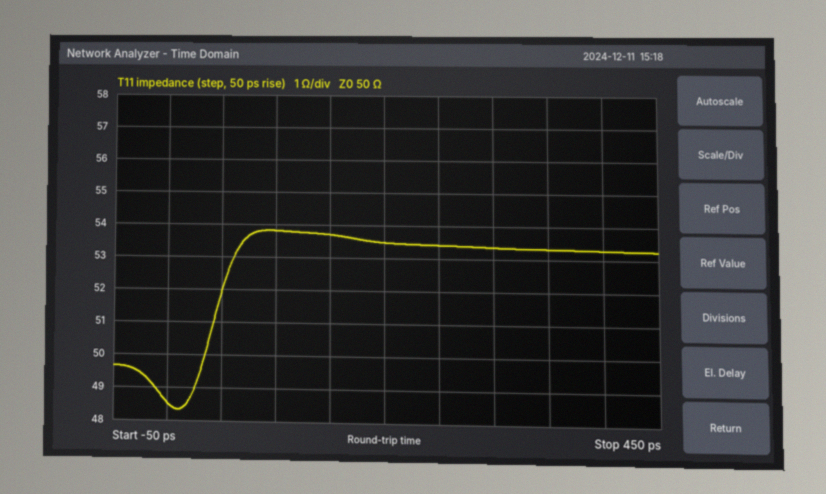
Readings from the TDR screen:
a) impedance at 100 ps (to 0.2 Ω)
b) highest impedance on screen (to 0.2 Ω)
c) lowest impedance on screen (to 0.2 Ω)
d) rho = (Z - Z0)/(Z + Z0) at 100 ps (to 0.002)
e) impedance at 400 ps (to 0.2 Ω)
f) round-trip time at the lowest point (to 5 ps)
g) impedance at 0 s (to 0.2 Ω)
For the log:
53.8 Ω
53.8 Ω
48.4 Ω
+0.036
53.2 Ω
10 ps
48.6 Ω
